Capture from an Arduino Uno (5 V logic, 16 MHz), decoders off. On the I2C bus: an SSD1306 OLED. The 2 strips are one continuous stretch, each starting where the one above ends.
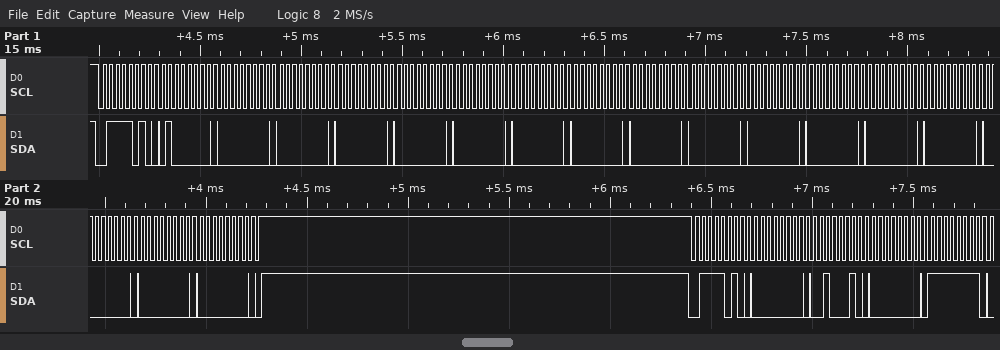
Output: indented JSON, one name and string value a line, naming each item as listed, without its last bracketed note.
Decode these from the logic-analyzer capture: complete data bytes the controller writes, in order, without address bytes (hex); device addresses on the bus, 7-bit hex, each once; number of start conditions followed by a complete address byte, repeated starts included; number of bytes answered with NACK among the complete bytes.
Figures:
{
  "complete data bytes the controller writes, in order, without address bytes": "40 00 00 00 00 00 00 00 00 00 00 00 00 00 00 00 00 00 22 00 FF",
  "device addresses on the bus, 7-bit hex, each once": "0x3D",
  "number of start conditions followed by a complete address byte, repeated starts included": "2",
  "number of bytes answered with NACK among the complete bytes": "0"
}
